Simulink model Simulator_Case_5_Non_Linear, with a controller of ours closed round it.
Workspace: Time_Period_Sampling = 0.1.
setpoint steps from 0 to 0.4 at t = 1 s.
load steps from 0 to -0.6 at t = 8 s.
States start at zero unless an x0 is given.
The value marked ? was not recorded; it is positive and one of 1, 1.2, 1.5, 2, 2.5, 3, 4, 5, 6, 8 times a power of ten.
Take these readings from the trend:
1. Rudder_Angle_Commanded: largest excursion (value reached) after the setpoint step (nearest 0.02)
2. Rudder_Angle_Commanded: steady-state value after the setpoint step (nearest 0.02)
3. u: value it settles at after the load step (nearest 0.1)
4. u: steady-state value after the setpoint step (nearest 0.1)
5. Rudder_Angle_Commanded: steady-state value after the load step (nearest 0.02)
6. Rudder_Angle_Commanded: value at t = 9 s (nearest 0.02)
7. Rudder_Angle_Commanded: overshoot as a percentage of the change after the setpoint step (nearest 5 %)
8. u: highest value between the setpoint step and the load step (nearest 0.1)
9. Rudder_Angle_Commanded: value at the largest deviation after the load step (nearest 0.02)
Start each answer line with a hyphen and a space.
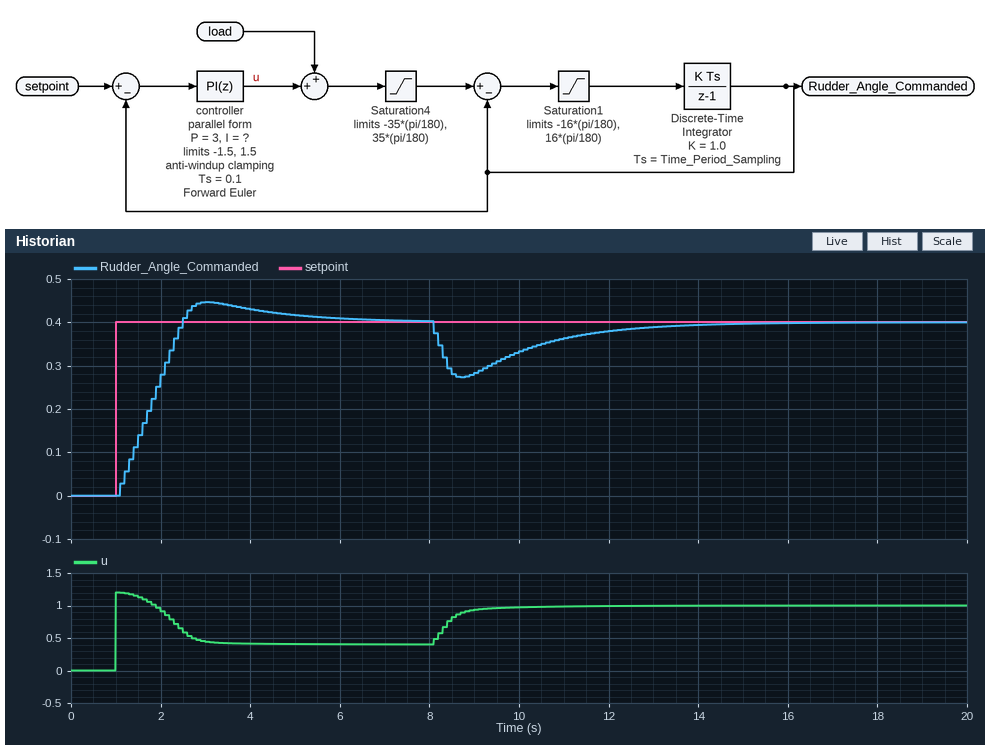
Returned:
- 0.44
- 0.40
- 1.0
- 0.4
- 0.40
- 0.28
- 10 %
- 1.2
- 0.28
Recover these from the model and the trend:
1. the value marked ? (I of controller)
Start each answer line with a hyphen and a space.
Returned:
- 2
